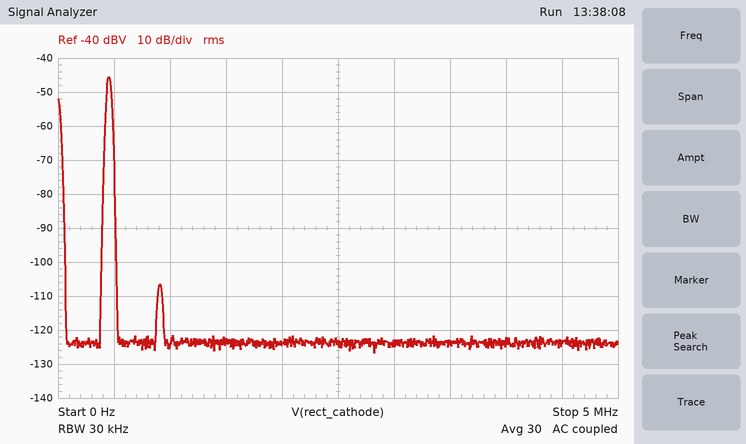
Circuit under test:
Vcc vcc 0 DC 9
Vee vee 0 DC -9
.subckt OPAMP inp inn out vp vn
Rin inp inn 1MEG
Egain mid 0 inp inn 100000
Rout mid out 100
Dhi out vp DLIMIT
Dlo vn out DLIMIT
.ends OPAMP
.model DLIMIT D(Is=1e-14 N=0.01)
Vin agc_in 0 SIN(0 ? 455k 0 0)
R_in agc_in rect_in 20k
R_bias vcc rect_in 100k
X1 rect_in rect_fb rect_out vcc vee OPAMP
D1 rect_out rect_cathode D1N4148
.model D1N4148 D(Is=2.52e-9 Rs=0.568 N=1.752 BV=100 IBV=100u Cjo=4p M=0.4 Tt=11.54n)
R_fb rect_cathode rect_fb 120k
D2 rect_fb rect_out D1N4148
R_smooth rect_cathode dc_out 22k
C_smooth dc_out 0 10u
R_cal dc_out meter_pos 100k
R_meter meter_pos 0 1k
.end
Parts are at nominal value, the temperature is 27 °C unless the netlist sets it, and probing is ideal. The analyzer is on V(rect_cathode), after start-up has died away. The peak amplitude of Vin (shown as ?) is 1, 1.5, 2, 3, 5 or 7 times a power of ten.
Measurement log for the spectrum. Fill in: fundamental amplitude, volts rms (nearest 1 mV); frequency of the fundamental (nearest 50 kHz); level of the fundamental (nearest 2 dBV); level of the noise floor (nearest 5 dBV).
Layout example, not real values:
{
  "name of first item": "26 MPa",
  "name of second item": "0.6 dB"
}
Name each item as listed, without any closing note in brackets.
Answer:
{
  "fundamental amplitude, volts rms": "5 mV",
  "frequency of the fundamental": "450 kHz",
  "level of the fundamental": "-46 dBV",
  "level of the noise floor": "-125 dBV"
}
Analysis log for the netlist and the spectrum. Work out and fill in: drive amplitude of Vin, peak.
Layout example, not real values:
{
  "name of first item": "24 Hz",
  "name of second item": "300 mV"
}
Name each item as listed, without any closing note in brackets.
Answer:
{
  "drive amplitude of Vin, peak": "10 mV"
}
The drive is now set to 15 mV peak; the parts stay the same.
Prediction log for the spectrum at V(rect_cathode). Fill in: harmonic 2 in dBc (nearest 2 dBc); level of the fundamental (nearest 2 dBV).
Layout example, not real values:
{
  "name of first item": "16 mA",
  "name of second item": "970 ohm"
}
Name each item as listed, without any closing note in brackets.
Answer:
{
  "harmonic 2 in dBc": "-58 dBc",
  "level of the fundamental": "-42 dBV"
}
